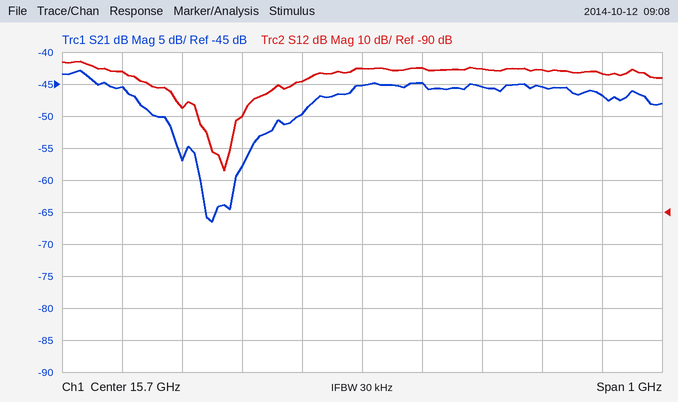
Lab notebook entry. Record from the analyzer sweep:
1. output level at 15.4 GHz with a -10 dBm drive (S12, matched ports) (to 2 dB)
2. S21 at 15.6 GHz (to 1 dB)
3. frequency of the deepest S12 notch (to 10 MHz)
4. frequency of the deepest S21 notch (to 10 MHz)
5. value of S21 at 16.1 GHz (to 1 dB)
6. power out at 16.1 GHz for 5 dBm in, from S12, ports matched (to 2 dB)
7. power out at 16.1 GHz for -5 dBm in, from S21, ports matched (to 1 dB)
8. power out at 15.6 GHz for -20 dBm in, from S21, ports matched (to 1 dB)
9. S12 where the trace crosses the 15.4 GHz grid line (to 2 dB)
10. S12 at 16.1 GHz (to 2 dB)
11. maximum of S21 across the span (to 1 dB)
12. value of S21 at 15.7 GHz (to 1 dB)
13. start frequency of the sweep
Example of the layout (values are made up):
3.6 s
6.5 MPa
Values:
-68 dBm
-50 dB
15.47 GHz
15.45 GHz
-47 dB
-42 dBm
-52 dBm
-70 dBm
-58 dB
-46 dB
-43 dB
-45 dB
15.2 GHz
